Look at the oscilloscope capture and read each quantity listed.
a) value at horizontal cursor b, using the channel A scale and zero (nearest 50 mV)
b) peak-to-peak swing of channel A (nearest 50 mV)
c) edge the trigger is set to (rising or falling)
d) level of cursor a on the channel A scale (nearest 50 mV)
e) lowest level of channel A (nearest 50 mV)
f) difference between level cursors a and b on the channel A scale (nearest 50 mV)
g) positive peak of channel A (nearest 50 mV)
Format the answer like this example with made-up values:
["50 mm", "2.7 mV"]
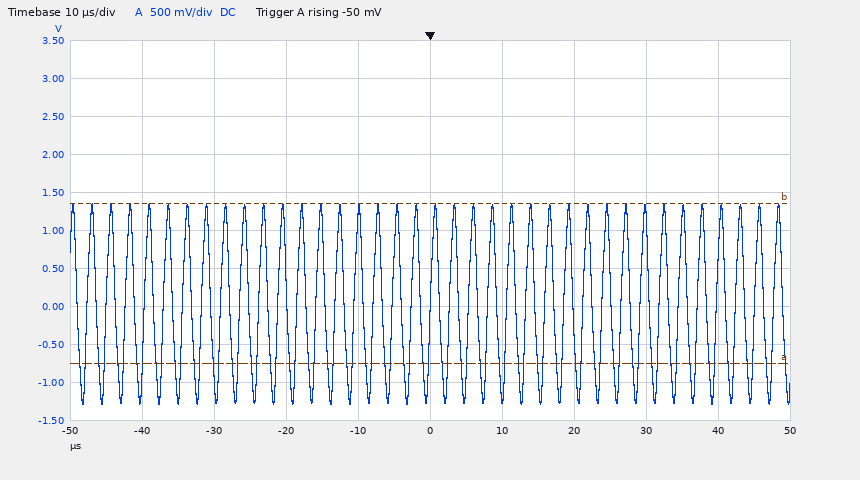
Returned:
["1.35 V", "2.65 V", "rising", "-750 mV", "-1.30 V", "2.10 V", "1.35 V"]
